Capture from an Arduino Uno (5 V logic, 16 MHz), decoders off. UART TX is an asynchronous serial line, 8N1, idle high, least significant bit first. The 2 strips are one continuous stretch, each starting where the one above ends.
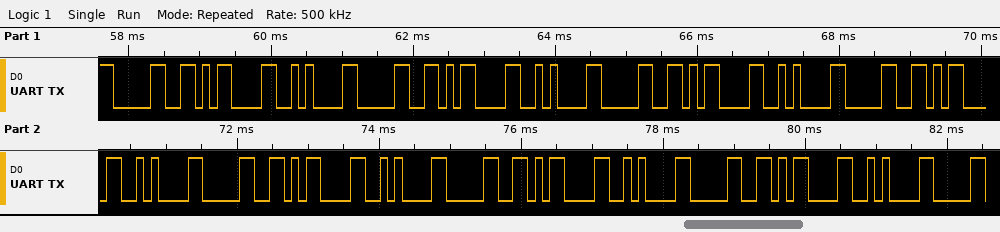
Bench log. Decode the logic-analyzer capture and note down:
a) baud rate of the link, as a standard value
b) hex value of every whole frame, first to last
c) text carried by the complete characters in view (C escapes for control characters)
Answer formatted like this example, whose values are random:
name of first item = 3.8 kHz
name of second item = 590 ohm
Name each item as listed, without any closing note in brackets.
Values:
baud rate of the link, as a standard value = 9600 baud
hex value of every whole frame, first to last = 30 0D 0A 30 0D 0A 30 0D 0A 30 0D 0A 30 0D 0A 30 0D 0A 30 0D 0A
text carried by the complete characters in view = "0\r\n0\r\n0\r\n0\r\n0\r\n0\r\n0\r\n"
